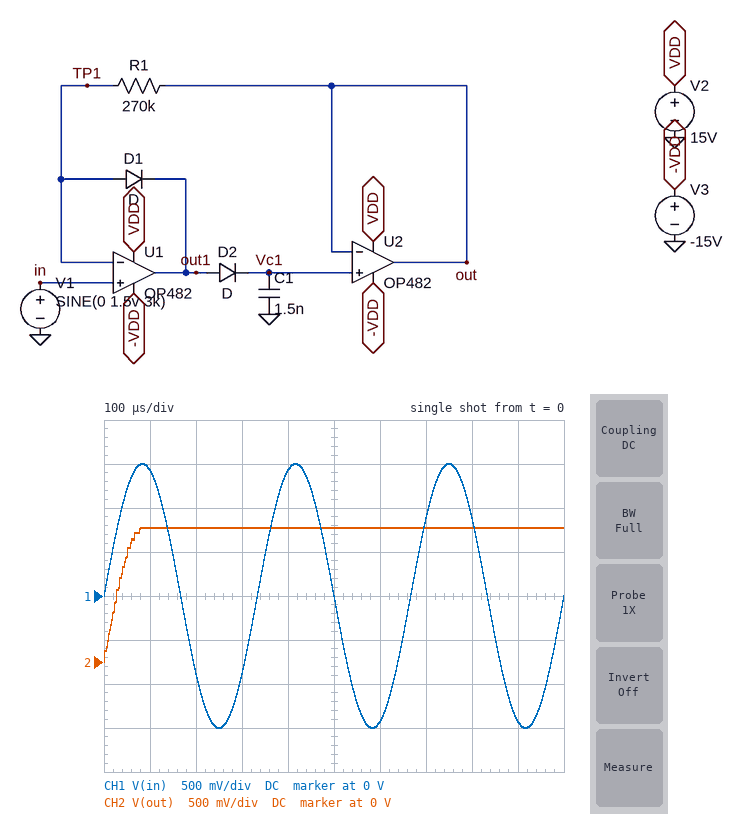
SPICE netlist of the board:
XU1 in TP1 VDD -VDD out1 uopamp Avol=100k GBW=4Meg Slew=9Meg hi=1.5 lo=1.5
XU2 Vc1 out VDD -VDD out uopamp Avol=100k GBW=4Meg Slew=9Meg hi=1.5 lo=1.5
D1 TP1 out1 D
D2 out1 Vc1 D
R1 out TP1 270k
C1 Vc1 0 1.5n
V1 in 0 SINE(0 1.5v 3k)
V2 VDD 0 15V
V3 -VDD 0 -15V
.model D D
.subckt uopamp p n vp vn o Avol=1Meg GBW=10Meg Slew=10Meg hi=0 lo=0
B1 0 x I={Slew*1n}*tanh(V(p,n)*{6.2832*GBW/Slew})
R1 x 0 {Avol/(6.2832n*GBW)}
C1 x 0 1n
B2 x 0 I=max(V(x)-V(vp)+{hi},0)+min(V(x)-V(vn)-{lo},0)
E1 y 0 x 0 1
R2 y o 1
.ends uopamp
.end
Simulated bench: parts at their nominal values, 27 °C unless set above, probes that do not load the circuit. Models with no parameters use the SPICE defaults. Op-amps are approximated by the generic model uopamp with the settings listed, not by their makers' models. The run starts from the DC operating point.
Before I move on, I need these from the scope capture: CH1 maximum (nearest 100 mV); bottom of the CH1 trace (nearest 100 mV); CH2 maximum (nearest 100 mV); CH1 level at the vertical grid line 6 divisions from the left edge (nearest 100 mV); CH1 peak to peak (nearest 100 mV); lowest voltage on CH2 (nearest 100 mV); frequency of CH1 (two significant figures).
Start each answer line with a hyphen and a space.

- 1.5 V
- -1.5 V
- 1.5 V
- -1.4 V
- 3.0 V
- 0 V
- 3.0 kHz
